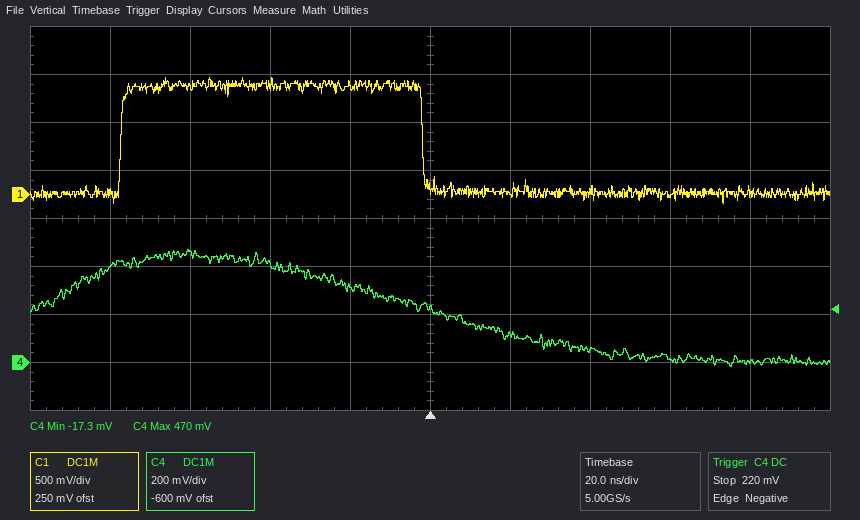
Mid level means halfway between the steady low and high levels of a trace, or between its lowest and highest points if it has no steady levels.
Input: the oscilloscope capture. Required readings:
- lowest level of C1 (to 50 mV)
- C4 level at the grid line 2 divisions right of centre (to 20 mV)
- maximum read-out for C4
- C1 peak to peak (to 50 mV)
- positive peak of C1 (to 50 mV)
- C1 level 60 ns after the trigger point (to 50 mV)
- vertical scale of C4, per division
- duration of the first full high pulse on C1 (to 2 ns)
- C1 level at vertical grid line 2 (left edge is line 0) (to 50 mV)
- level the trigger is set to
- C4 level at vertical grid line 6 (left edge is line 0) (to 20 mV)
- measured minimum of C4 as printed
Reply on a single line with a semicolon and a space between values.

-100 mV; 60 mV; 470 mV; 1.30 V; 1.20 V; 0 mV; 200 mV; 76 ns; 1.15 V; 220 mV; 120 mV; -17.3 mV
